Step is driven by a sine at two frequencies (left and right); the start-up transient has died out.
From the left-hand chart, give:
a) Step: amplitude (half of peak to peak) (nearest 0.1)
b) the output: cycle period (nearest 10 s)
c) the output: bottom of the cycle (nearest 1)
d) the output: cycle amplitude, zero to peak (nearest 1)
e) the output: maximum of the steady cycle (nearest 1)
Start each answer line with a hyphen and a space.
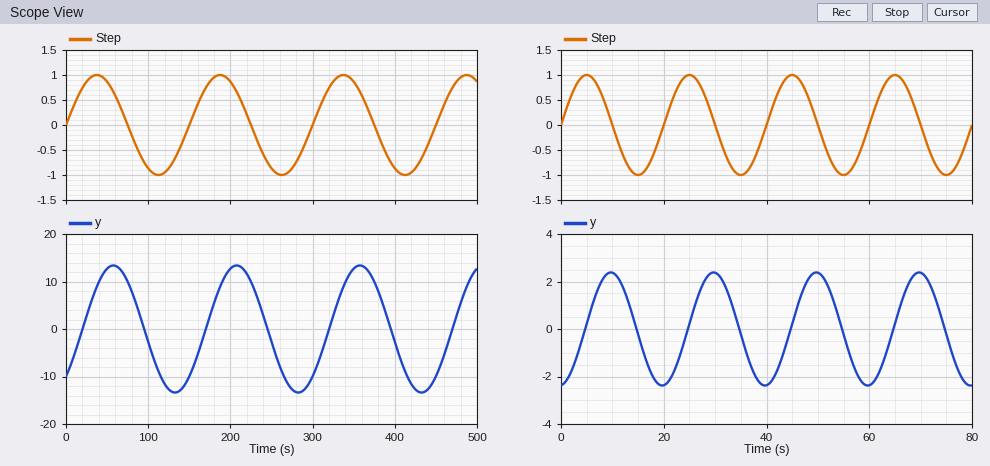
- 1.0
- 150 s
- -13
- 13
- 13
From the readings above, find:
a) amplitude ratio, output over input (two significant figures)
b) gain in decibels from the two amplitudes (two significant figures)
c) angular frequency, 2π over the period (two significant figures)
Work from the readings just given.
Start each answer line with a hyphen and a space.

- 13
- 22 dB
- 0.042 rad/s
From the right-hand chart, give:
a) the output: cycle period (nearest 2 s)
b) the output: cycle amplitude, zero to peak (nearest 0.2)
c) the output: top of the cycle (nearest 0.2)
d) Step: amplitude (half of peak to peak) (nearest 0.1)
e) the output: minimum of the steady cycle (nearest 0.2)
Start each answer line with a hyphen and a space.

- 20 s
- 2.4
- 2.4
- 1.0
- -2.4
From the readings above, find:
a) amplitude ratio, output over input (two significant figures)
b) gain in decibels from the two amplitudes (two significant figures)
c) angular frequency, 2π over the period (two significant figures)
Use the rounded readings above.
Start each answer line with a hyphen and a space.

- 2.4
- 7.6 dB
- 0.31 rad/s
